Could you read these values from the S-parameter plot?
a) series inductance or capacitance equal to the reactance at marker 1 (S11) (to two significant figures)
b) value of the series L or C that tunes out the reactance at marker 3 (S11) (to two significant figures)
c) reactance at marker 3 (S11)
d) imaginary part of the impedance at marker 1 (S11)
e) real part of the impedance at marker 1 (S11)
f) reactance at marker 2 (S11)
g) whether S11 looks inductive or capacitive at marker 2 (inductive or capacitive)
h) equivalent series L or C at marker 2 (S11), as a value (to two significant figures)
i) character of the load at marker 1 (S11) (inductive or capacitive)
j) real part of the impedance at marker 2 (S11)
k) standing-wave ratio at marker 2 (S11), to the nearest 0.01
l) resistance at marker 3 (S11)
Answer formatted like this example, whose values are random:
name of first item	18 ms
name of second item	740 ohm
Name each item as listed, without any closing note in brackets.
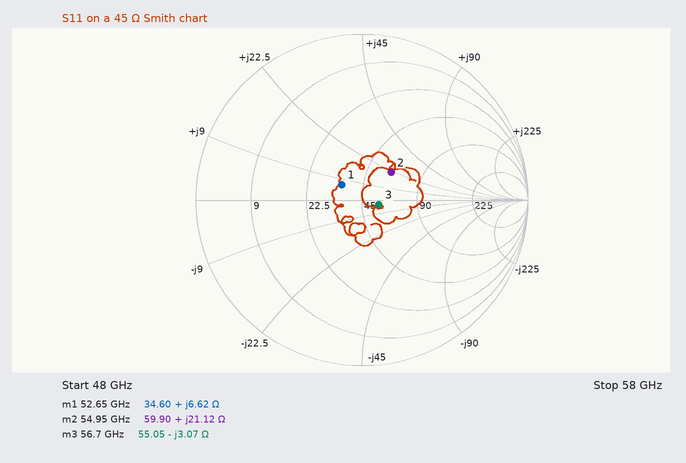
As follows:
series inductance or capacitance equal to the reactance at marker 1 (S11)	20 pH
value of the series L or C that tunes out the reactance at marker 3 (S11)	8.6 pH
reactance at marker 3	-3.07 Ω
imaginary part of the impedance at marker 1	+6.62 Ω
real part of the impedance at marker 1	34.60 Ω
reactance at marker 2	+21.12 Ω
whether S11 looks inductive or capacitive at marker 2	inductive
equivalent series L or C at marker 2 (S11), as a value	61 pH
character of the load at marker 1 (S11)	inductive
real part of the impedance at marker 2	59.90 Ω
standing-wave ratio at marker 2 (S11), to the nearest 0.01	1.64
resistance at marker 3	55.05 Ω
